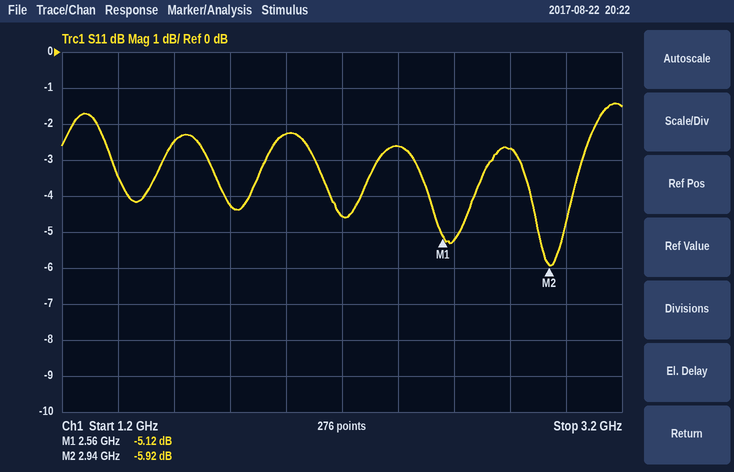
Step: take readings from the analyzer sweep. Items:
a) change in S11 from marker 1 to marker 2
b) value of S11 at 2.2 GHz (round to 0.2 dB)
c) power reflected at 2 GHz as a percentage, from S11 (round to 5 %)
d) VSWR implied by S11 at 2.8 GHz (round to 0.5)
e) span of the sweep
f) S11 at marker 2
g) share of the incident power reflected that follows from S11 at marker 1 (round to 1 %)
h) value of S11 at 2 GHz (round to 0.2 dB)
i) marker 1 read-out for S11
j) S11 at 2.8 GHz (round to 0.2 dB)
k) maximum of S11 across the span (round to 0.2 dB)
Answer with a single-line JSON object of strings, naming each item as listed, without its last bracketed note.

{"change in S11 from marker 1 to marker 2": "-0.80 dB", "value of S11 at 2.2 GHz": "-4.6 dB", "power reflected at 2 GHz as a percentage, from S11": "60 %", "VSWR implied by S11 at 2.8 GHz": "6.5", "span of the sweep": "2 GHz", "S11 at marker 2": "-5.92 dB", "share of the incident power reflected that follows from S11 at marker 1": "31 %", "value of S11 at 2 GHz": "-2.2 dB", "marker 1 read-out for S11": "-5.12 dB", "S11 at 2.8 GHz": "-2.6 dB", "maximum of S11 across the span": "-1.4 dB"}
